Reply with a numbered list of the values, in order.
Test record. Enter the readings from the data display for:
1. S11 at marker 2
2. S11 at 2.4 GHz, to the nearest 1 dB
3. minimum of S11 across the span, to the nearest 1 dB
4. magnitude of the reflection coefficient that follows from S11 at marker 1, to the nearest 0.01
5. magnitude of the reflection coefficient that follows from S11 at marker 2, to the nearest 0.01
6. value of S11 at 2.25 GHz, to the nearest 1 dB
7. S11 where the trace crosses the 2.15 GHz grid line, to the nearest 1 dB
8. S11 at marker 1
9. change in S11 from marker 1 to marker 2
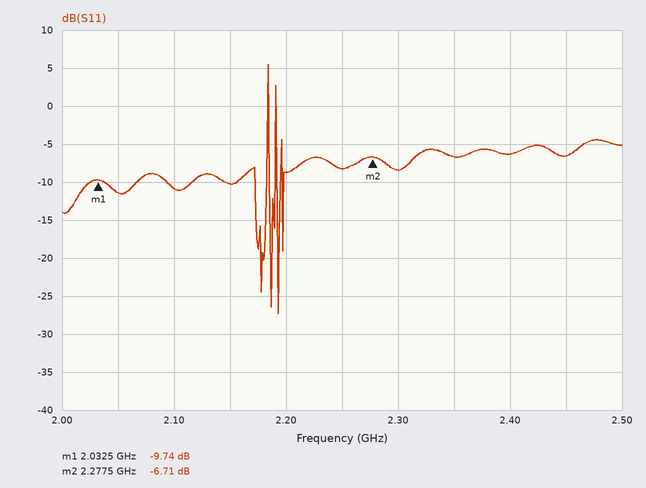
1. -6.71 dB
2. -6 dB
3. -27 dB
4. 0.33
5. 0.46
6. -8 dB
7. -10 dB
8. -9.74 dB
9. 3.03 dB
